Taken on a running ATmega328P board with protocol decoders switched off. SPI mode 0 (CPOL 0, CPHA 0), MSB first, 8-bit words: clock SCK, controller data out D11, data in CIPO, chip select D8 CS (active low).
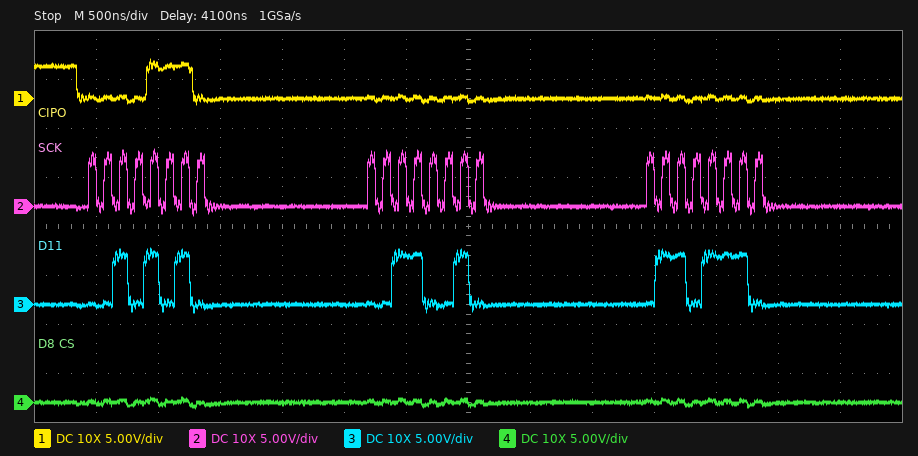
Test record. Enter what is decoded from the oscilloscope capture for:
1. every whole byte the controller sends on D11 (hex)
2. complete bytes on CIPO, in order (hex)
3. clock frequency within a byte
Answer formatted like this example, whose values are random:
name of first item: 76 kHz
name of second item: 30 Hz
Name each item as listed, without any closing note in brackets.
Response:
every whole byte the controller sends on D11: 2A 32 6E
complete bytes on CIPO, in order: 0E 00 00
clock frequency within a byte: 8 MHz
